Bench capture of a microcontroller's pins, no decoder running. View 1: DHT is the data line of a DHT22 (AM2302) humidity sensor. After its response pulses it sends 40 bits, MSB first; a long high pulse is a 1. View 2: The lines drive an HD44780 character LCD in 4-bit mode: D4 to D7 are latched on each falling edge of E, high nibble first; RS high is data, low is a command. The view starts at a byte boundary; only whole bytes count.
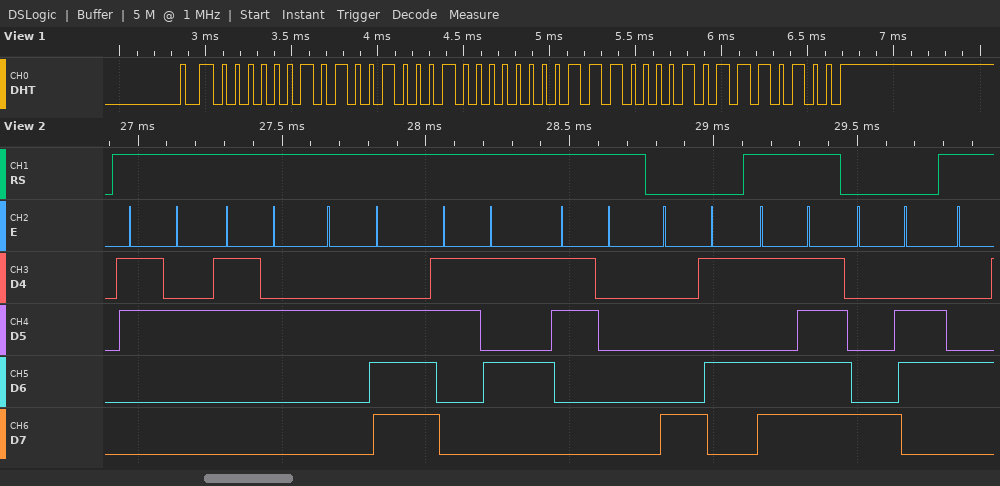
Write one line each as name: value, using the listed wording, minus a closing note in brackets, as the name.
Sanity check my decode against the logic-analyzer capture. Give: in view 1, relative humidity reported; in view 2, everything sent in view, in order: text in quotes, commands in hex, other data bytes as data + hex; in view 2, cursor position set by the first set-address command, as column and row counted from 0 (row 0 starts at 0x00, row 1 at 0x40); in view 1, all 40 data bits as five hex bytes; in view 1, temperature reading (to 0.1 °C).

in view 1, relative humidity reported: 65.7 %
in view 2, everything sent in view, in order: text in quotes, commands in hex, other data bytes as data + hex: "22.50" 0x85 data DF 0x86
in view 2, cursor position set by the first set-address command, as column and row counted from 0: column 5, row 0
in view 1, all 40 data bits as five hex bytes: 02 91 00 E1 74
in view 1, temperature reading: 22.5 °C
